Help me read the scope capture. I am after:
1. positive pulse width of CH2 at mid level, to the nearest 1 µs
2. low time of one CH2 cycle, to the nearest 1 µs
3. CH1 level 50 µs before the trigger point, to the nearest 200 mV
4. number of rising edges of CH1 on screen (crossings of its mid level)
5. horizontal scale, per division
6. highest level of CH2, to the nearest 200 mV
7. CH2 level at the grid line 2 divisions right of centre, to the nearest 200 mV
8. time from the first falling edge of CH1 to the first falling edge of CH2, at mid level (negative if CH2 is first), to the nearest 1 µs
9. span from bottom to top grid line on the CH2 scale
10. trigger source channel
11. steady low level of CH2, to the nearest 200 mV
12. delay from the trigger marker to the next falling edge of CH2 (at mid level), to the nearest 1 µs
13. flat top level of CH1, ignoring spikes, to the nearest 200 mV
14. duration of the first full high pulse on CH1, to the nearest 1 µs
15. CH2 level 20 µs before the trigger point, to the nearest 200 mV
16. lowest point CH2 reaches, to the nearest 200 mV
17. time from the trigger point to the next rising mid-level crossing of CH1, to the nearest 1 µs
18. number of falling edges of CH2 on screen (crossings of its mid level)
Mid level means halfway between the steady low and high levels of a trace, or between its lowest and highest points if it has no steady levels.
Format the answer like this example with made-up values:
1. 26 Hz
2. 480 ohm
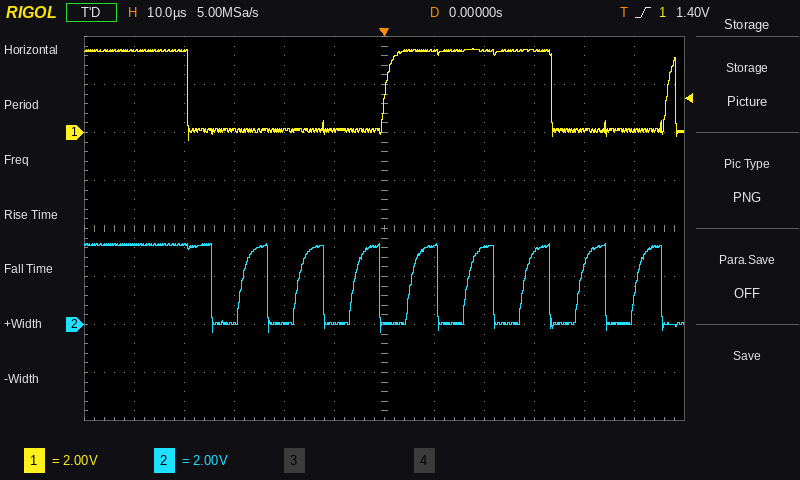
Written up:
1. 5 µs
2. 6 µs
3. 3.4 V
4. 2
5. 10 µs
6. 3.4 V
7. 3.2 V
8. +5 µs
9. 16 V
10. CH1
11. 0.0 V
12. 11 µs
13. 3.4 V
14. 33 µs
15. 0.0 V
16. -400 mV
17. 57 µs
18. 9
